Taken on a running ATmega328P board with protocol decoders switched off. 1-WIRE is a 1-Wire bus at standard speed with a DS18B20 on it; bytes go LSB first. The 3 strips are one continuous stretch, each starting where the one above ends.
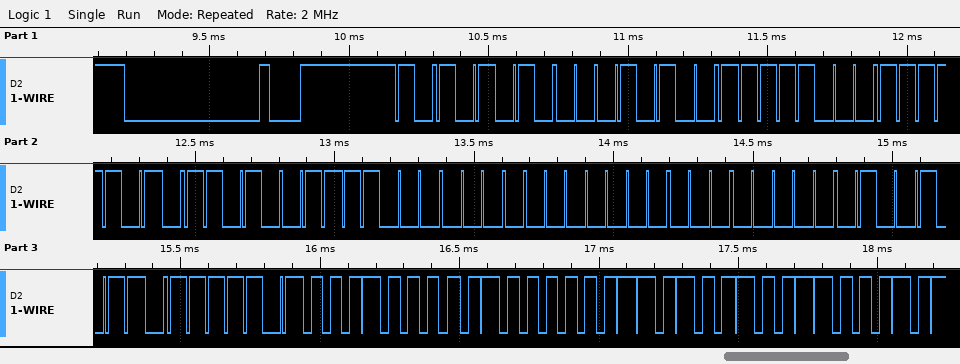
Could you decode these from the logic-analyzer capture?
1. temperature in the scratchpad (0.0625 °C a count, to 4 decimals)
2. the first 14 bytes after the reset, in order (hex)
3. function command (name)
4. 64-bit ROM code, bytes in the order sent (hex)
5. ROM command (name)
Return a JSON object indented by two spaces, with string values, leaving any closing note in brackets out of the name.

{
  "temperature in the scratchpad": "32.5000 °C",
  "the first 14 bytes after the reset, in order": "55 28 1F 5F CB 03 00 00 D2 BE 08 02 4B 46",
  "function command": "Read Scratchpad",
  "64-bit ROM code, bytes in the order sent": "28 1F 5F CB 03 00 00 D2",
  "ROM command": "Match ROM"
}
